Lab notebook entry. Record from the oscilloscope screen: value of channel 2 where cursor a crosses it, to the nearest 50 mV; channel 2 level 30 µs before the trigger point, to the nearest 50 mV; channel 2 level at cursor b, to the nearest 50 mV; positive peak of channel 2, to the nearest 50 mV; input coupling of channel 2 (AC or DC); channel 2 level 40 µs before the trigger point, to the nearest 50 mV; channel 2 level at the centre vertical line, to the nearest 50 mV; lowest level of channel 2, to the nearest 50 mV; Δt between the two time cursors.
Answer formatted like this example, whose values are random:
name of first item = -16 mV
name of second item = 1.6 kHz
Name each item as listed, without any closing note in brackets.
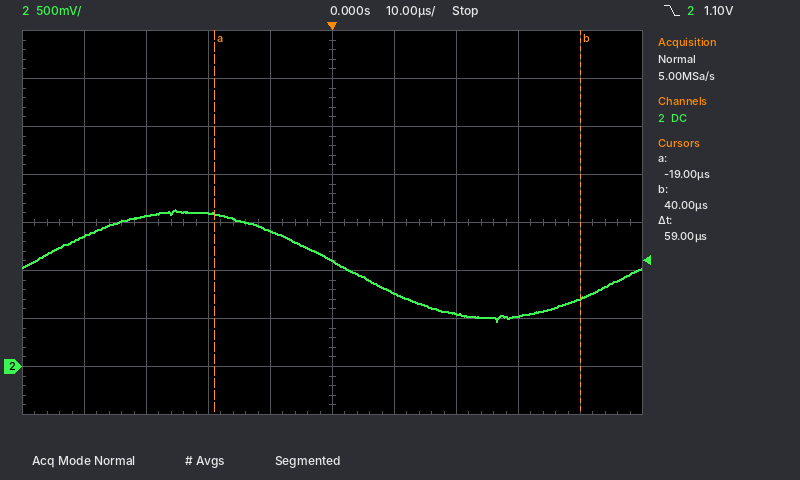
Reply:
value of channel 2 where cursor a crosses it, to the nearest 50 mV = 1.60 V
channel 2 level 30 µs before the trigger point, to the nearest 50 mV = 1.55 V
channel 2 level at cursor b, to the nearest 50 mV = 700 mV
positive peak of channel 2, to the nearest 50 mV = 1.65 V
input coupling of channel 2 = DC
channel 2 level 40 µs before the trigger point, to the nearest 50 mV = 1.35 V
channel 2 level at the centre vertical line, to the nearest 50 mV = 1.10 V
lowest level of channel 2, to the nearest 50 mV = 450 mV
Δt between the two time cursors = 59 µs
